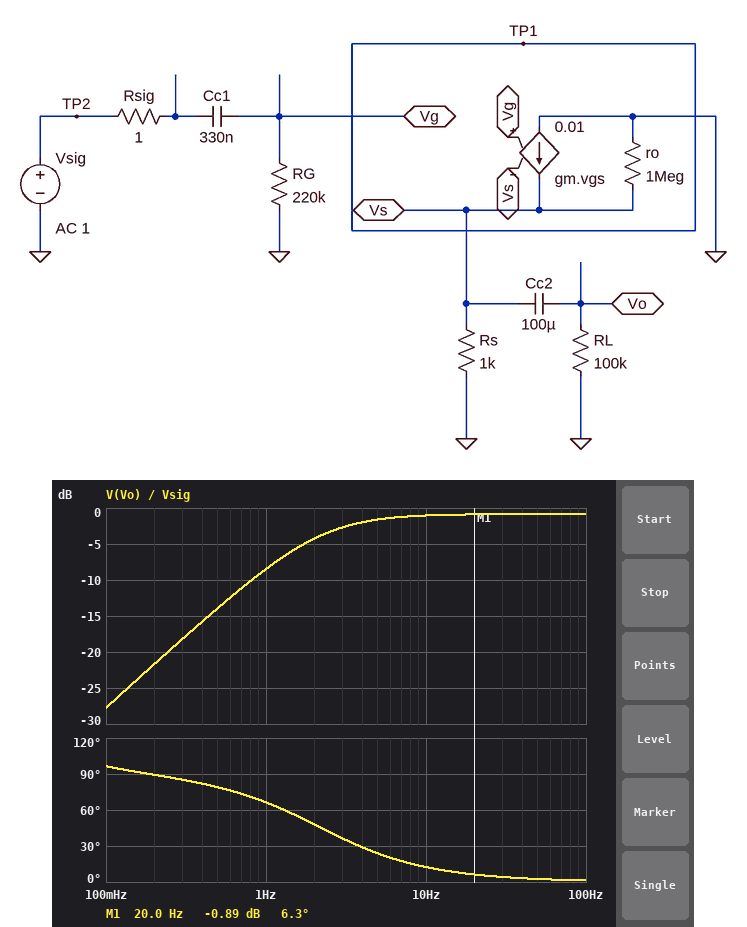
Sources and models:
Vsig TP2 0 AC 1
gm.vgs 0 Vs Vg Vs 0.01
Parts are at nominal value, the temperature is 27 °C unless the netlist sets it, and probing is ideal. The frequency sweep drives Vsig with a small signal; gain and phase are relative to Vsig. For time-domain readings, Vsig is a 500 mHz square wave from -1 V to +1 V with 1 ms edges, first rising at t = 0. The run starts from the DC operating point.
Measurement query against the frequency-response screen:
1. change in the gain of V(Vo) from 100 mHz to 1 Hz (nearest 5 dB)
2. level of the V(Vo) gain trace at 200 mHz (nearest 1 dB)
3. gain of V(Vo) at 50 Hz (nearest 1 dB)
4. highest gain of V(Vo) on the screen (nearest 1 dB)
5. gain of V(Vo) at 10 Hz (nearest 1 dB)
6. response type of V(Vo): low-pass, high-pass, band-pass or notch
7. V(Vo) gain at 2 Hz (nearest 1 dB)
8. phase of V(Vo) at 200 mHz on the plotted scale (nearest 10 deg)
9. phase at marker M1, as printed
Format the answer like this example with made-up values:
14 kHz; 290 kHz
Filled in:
20 dB; -22 dB; -1 dB; -1 dB; -1 dB; high-pass; -4 dB; 90 deg; 6.3 deg
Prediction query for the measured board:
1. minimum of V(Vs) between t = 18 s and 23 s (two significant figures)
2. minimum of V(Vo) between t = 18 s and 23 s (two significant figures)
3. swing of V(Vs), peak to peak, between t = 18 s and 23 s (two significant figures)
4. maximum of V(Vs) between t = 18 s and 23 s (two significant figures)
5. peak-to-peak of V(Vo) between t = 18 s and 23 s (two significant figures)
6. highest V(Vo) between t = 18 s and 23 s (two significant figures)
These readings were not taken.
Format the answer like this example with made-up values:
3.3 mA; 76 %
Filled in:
-1.8 V; -1.8 V; 3.6 V; 1.8 V; 3.6 V; 1.8 V
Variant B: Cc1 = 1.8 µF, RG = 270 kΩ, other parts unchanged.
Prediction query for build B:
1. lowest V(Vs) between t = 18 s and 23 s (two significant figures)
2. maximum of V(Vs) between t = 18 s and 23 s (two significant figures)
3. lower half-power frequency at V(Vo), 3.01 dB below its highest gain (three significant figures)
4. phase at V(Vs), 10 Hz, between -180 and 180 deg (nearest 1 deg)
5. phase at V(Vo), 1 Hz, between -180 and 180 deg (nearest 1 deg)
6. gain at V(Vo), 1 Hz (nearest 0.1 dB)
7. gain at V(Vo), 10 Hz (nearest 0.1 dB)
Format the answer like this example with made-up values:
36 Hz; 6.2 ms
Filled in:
-1.6 V; 1.6 V; 328 mHz; 2 deg; 19 deg; -1.3 dB; -0.8 dB
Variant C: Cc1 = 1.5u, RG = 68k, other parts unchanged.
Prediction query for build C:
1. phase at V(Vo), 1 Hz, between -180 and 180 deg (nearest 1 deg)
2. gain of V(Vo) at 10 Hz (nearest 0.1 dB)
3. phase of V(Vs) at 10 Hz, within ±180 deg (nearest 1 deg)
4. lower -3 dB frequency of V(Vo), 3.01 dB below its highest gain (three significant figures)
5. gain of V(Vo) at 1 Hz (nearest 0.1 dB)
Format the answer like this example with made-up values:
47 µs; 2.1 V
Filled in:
58 deg; -0.9 dB; 9 deg; 1.56 Hz; -6.2 dB
